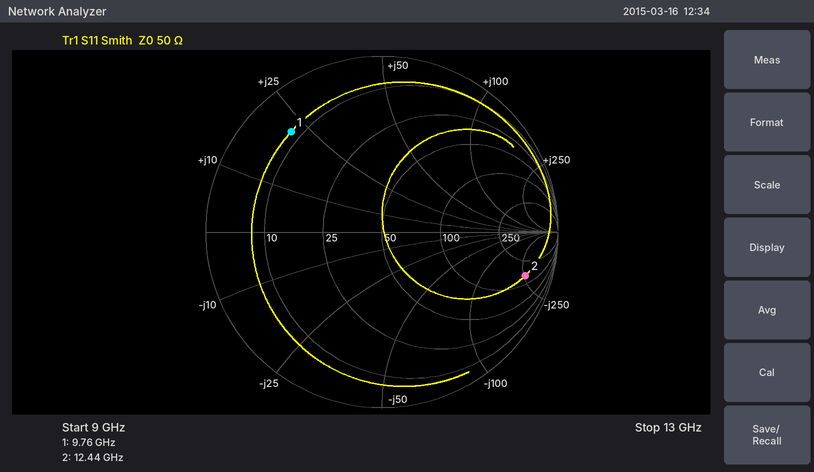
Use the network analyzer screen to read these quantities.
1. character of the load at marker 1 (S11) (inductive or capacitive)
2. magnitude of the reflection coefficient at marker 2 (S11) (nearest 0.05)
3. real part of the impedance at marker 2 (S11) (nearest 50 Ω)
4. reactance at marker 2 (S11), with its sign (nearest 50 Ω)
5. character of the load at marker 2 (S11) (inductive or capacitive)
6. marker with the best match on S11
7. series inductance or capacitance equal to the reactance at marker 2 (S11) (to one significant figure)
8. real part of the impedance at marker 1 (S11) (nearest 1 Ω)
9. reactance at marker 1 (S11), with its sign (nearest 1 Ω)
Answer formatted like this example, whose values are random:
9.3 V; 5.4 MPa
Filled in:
inductive; 0.85; 150 Ω; -250 Ω; capacitive; marker 1; 50 fF; 8 Ω; +22 Ω
